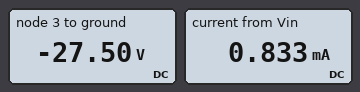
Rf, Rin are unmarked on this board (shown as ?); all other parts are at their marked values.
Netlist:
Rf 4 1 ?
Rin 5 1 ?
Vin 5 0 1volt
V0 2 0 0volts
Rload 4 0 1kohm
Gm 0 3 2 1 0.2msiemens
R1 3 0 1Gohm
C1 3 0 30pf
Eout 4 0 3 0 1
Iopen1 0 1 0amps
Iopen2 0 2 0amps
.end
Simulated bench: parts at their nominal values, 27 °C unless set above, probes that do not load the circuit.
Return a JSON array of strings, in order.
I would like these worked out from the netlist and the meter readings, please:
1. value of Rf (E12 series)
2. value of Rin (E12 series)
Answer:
["33 kΩ", "1.2 kΩ"]
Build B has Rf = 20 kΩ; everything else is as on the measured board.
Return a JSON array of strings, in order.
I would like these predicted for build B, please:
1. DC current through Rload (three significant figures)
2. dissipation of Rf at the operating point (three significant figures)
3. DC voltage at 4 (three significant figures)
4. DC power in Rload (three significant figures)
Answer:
["16.7 mA", "13.9 mW", "-16.7 V", "278 mW"]
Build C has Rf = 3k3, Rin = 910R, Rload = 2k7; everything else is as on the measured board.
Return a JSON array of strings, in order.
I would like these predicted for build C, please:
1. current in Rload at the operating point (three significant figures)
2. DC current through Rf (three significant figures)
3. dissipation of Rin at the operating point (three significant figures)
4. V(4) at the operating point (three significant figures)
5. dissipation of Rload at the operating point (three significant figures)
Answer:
["1.34 mA", "1.10 mA", "1.10 mW", "-3.63 V", "4.87 mW"]
